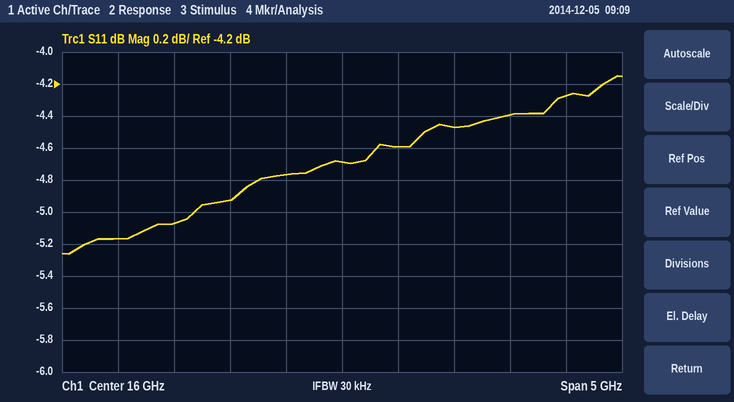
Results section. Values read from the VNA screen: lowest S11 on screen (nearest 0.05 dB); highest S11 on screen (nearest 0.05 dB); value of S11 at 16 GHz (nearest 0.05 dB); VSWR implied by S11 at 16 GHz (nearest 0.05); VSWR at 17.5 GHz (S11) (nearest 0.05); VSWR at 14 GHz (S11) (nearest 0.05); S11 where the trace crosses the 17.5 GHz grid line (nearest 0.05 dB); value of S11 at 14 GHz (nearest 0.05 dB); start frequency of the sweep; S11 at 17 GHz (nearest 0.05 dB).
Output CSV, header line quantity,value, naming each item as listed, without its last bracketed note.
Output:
quantity,value
lowest S11 on screen,-5.25 dB
highest S11 on screen,-4.15 dB
value of S11 at 16 GHz,-4.70 dB
VSWR implied by S11 at 16 GHz,3.80
VSWR at 17.5 GHz (S11),4.05
VSWR at 14 GHz (S11),3.45
S11 where the trace crosses the 17.5 GHz grid line,-4.40 dB
value of S11 at 14 GHz,-5.15 dB
start frequency of the sweep,13.5 GHz
S11 at 17 GHz,-4.45 dB
